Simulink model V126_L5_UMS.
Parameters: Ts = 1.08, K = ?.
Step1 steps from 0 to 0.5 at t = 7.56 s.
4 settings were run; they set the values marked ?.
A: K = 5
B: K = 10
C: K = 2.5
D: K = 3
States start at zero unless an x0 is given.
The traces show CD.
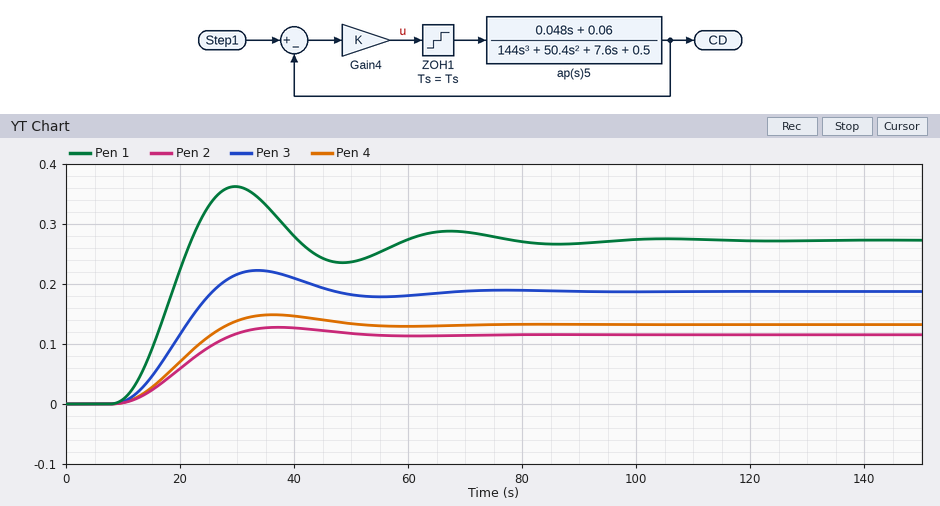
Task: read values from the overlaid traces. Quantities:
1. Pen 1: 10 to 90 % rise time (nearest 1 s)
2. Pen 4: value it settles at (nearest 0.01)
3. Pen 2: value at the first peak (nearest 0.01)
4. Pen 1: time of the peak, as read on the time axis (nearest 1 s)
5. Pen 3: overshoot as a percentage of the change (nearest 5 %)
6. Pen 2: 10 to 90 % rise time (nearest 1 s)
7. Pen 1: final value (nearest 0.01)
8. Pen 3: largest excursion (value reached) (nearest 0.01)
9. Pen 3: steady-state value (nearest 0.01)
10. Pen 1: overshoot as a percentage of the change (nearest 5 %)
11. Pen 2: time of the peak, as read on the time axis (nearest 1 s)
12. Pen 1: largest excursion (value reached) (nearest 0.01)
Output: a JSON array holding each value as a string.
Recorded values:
["9 s", "0.13", "0.13", "30 s", "20 %", "14 s", "0.27", "0.22", "0.19", "35 %", "37 s", "0.36"]
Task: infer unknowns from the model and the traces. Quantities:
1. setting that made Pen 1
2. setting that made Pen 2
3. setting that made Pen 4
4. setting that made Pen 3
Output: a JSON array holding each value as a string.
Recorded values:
["B", "C", "D", "A"]
